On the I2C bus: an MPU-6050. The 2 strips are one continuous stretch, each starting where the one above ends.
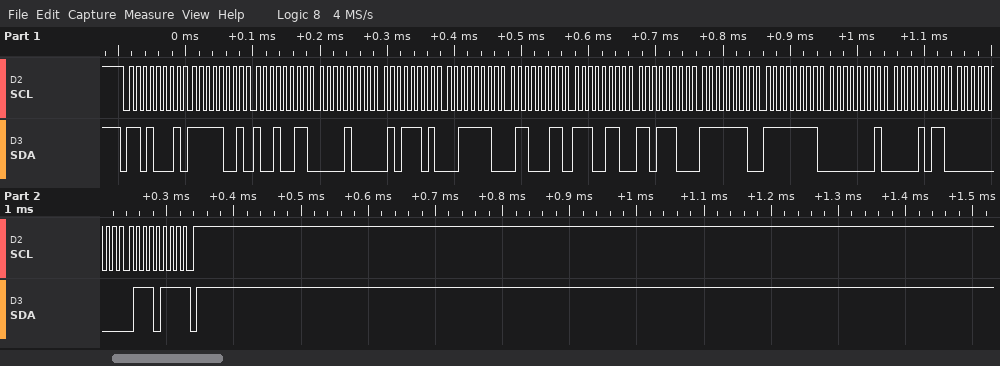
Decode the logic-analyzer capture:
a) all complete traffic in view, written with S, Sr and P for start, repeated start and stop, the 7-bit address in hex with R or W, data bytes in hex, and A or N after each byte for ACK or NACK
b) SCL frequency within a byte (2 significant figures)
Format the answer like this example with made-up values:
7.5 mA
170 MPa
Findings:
S 68R A F9 A 93 A 08 A 5D A 3E A 63 A E6 A DC A FE A FF A 01 A 0B A 00 A 77 N P
100 kHz
